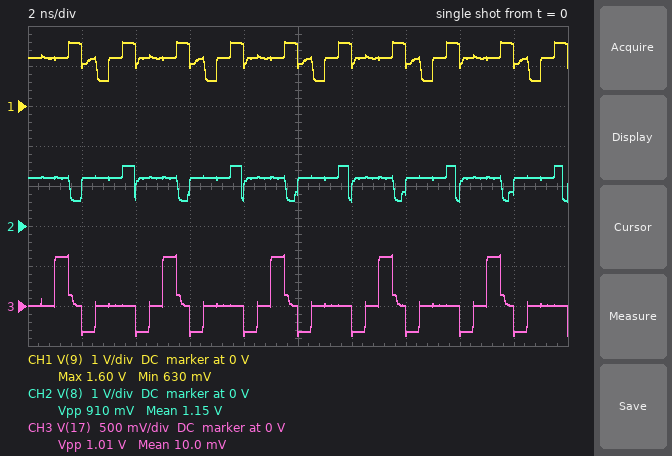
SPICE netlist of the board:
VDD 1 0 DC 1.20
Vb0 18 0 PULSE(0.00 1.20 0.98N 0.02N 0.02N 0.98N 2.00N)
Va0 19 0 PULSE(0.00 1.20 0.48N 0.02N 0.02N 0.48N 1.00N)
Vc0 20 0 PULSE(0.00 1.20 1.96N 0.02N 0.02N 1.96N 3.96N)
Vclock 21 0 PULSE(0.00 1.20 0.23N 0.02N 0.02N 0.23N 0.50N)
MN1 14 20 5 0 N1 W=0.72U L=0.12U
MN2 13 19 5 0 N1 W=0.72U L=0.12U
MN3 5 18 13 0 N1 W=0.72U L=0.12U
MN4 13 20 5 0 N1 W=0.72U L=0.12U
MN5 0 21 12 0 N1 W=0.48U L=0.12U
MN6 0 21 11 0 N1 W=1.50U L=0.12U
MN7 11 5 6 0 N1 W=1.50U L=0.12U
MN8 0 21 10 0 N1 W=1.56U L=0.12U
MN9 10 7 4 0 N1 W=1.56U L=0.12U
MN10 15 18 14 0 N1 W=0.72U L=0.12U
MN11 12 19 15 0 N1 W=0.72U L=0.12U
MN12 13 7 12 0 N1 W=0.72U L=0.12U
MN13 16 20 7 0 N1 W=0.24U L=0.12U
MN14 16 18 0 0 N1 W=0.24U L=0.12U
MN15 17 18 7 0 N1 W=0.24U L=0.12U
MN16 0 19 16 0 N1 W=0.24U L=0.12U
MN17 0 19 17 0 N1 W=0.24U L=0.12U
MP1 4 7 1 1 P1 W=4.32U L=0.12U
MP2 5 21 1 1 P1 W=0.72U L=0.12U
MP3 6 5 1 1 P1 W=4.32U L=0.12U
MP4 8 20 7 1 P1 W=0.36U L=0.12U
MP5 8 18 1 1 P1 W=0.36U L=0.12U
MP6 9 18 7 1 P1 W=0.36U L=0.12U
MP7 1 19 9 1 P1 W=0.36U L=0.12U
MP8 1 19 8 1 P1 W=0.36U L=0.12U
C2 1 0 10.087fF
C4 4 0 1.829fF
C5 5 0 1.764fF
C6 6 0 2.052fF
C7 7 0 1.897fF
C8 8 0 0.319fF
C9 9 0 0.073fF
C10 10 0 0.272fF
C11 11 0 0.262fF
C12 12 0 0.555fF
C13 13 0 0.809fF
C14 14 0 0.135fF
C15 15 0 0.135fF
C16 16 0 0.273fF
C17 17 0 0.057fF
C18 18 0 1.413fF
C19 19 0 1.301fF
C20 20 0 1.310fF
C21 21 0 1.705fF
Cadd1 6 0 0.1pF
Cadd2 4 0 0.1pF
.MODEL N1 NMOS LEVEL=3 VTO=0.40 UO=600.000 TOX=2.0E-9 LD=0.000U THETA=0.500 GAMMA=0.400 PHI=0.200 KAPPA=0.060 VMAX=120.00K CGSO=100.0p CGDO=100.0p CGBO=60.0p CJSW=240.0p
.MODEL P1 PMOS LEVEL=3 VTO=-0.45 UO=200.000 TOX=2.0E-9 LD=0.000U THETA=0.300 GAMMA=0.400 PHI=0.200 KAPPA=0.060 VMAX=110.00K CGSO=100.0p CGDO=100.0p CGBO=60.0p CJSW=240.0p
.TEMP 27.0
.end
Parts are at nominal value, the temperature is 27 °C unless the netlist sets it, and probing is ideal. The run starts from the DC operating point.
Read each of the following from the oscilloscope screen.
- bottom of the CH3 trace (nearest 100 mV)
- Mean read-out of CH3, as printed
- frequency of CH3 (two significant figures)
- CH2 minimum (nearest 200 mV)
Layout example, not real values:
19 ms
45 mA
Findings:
-400 mV
10.0 mV
250 MHz
600 mV
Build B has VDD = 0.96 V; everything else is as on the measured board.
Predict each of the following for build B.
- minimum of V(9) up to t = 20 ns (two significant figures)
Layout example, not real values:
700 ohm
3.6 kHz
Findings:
580 mV
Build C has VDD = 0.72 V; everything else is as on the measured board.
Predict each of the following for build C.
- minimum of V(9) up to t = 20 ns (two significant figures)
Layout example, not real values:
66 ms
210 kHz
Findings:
520 mV
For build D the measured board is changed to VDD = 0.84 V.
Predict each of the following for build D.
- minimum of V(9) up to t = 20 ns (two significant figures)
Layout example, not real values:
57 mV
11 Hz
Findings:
550 mV
